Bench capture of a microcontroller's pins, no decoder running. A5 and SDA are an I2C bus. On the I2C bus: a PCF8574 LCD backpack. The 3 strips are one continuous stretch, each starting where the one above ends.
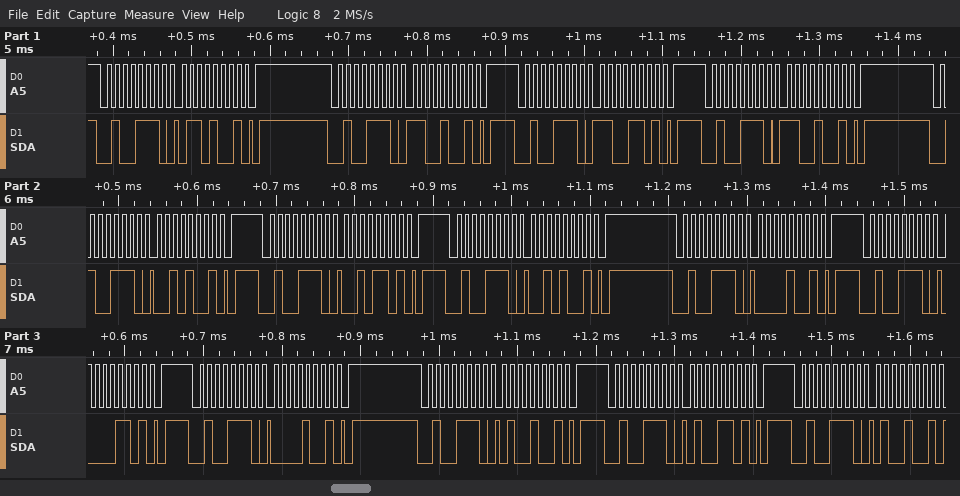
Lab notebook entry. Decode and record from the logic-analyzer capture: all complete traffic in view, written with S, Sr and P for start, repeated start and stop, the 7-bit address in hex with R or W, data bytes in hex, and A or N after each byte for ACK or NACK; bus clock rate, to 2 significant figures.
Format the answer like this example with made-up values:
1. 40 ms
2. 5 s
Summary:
1. S 27W A 69 A P S 27W A C9 A P S 27W A CD A P S 27W A C9 A P S 27W A 29 A P S 27W A 2D A P S 27W A 29 A P S 27W A 09 A P S 27W A 0D A P S 27W A 09 A P S 27W A 49 A P S 27W A 4D A P S 27W A 49 A
2. 100 kHz
